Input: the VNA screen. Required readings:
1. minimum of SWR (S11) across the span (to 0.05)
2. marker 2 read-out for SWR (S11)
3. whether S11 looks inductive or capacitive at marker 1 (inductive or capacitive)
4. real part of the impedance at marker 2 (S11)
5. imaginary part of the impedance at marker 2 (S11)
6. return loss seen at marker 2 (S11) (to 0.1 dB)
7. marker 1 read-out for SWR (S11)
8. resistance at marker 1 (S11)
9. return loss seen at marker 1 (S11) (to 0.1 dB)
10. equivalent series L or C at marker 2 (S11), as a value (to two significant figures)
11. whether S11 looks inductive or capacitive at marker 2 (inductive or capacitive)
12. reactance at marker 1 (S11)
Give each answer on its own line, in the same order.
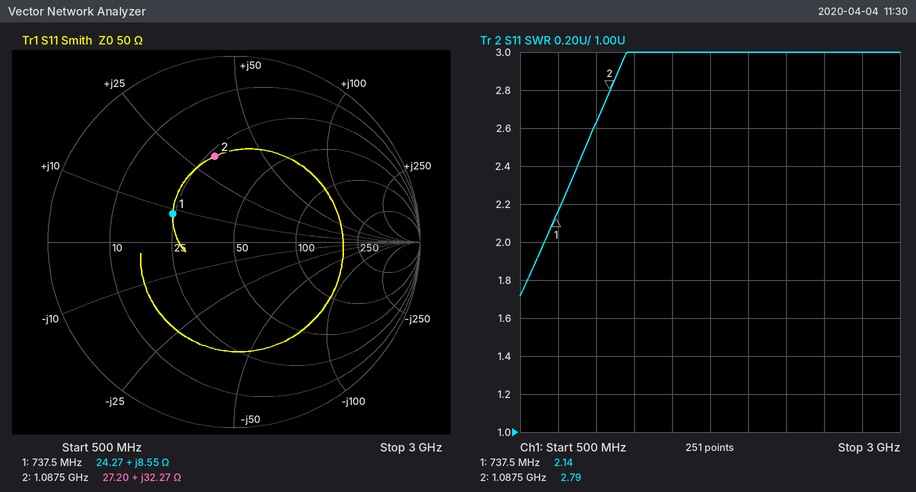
1.70
2.79
inductive
27.20 Ω
+32.27 Ω
6.5 dB
2.14
24.27 Ω
8.8 dB
4.7 nH
inductive
+8.55 Ω
